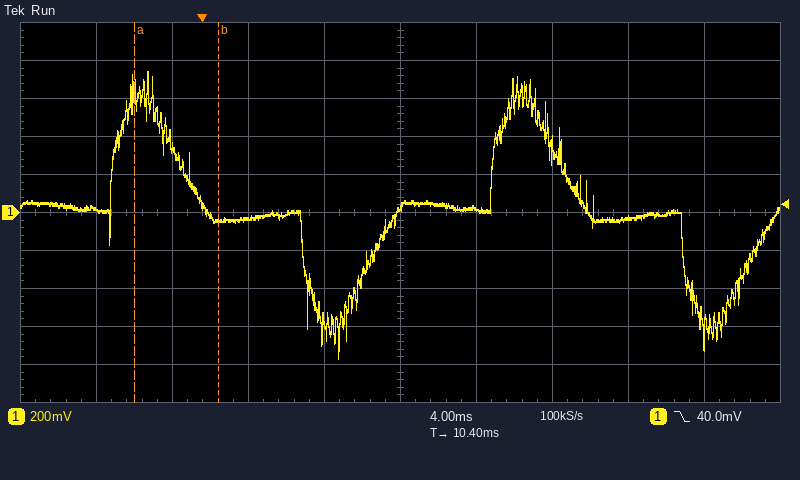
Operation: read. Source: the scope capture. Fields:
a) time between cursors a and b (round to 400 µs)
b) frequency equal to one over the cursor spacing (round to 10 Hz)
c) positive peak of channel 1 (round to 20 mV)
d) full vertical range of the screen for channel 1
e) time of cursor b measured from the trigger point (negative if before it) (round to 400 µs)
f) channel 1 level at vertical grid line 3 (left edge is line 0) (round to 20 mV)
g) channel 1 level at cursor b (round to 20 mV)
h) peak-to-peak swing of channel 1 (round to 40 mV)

4.4 ms
230 Hz
740 mV
2 V
+800 µs
-20 mV
-40 mV
1.52 V
